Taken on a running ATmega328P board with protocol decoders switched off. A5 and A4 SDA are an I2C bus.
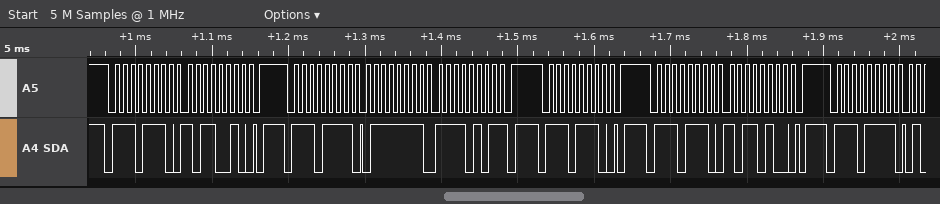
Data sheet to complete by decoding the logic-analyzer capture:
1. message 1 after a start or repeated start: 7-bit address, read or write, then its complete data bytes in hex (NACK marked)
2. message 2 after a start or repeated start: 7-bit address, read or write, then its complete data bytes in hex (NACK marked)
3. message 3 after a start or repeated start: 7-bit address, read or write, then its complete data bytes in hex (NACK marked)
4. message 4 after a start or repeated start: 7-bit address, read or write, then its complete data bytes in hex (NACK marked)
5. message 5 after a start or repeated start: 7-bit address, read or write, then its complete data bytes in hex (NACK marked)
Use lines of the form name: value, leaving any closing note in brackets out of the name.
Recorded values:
message 1 after a start or repeated start: 7-bit address, read or write, then its complete data bytes in hex: 0x77 write: B2
message 2 after a start or repeated start: 7-bit address, read or write, then its complete data bytes in hex: 0x77 read: 7F F5 NACK
message 3 after a start or repeated start: 7-bit address, read or write, then its complete data bytes in hex: 0x77 write
message 4 after a start or repeated start: 7-bit address, read or write, then its complete data bytes in hex: 0x77 write: B4
message 5 after a start or repeated start: 7-bit address, read or write, then its complete data bytes in hex: 0x77 read
